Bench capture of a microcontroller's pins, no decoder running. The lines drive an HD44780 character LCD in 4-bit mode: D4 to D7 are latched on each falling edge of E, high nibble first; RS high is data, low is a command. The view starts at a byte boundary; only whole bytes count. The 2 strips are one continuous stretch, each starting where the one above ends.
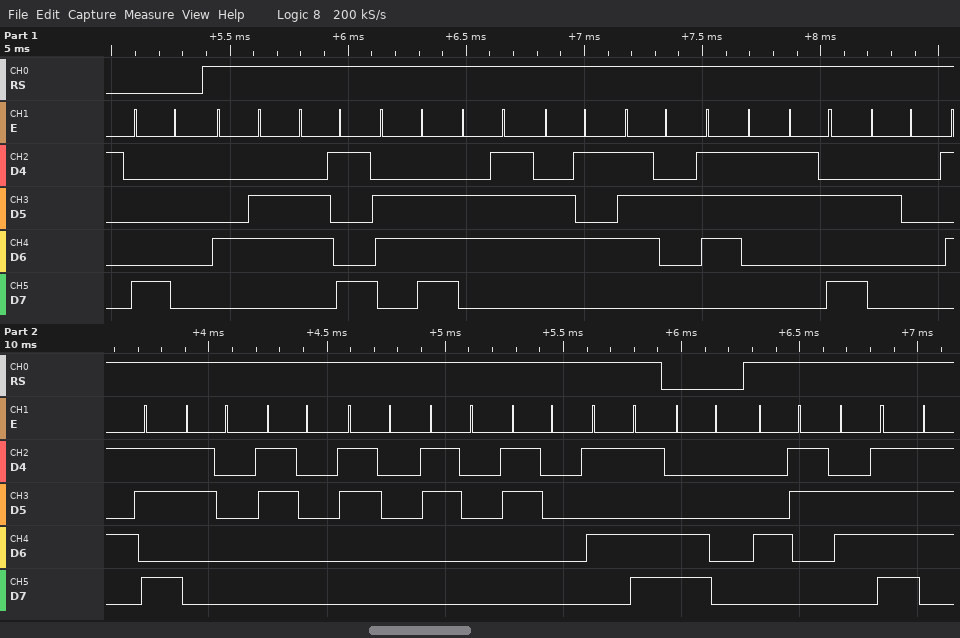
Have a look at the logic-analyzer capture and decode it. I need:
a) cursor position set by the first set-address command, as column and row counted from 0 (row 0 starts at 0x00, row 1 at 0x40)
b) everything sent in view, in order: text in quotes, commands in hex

column 0, row 0
0x80 "Fingers: [00000]" 0xC0 "Co"
